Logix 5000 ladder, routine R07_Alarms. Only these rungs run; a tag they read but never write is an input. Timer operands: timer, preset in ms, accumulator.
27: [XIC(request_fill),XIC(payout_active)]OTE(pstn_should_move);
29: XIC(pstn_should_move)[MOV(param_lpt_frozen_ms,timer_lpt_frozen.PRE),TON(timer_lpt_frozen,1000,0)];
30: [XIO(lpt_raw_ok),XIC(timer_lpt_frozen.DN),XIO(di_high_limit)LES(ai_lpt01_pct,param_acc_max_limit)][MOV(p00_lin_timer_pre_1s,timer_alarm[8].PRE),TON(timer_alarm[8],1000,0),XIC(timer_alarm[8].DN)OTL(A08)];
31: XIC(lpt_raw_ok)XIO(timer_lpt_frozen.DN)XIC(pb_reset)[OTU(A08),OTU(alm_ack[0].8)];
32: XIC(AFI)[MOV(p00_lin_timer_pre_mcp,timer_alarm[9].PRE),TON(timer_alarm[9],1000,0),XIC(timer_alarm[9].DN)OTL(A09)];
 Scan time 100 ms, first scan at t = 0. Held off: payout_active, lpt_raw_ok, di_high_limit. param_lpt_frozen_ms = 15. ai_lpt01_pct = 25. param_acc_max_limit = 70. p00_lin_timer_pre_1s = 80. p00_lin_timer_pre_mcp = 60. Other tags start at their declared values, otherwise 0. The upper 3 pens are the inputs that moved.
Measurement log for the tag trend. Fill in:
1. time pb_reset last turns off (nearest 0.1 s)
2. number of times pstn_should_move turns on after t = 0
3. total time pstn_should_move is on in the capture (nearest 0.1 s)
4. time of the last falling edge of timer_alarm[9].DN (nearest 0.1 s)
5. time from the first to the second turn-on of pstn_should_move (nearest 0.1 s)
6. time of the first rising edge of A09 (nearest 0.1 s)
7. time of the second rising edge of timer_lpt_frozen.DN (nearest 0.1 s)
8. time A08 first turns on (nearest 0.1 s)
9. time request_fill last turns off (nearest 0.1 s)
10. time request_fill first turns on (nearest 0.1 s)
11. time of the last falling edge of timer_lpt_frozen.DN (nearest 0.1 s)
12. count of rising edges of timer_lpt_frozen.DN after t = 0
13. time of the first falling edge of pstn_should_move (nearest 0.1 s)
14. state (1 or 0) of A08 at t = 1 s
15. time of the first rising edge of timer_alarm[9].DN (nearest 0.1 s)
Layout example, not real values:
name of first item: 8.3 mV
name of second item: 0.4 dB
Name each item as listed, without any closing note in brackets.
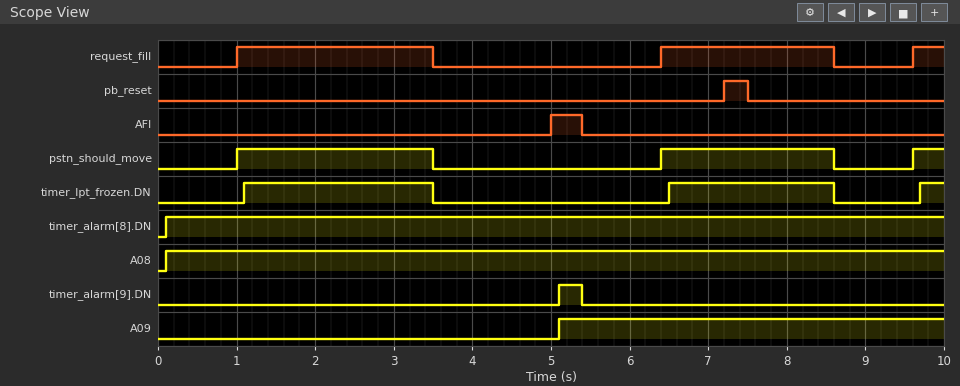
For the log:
time pb_reset last turns off: 7.5 s
number of times pstn_should_move turns on after t = 0: 3
total time pstn_should_move is on in the capture: 5.1 s
time of the last falling edge of timer_alarm[9].DN: 5.4 s
time from the first to the second turn-on of pstn_should_move: 5.4 s
time of the first rising edge of A09: 5.1 s
time of the second rising edge of timer_lpt_frozen.DN: 6.5 s
time A08 first turns on: 0.1 s
time request_fill last turns off: 8.6 s
time request_fill first turns on: 1.0 s
time of the last falling edge of timer_lpt_frozen.DN: 8.6 s
count of rising edges of timer_lpt_frozen.DN after t = 0: 3
time of the first falling edge of pstn_should_move: 3.5 s
state (1 or 0) of A08 at t = 1 s: 1
time of the first rising edge of timer_alarm[9].DN: 5.1 s
